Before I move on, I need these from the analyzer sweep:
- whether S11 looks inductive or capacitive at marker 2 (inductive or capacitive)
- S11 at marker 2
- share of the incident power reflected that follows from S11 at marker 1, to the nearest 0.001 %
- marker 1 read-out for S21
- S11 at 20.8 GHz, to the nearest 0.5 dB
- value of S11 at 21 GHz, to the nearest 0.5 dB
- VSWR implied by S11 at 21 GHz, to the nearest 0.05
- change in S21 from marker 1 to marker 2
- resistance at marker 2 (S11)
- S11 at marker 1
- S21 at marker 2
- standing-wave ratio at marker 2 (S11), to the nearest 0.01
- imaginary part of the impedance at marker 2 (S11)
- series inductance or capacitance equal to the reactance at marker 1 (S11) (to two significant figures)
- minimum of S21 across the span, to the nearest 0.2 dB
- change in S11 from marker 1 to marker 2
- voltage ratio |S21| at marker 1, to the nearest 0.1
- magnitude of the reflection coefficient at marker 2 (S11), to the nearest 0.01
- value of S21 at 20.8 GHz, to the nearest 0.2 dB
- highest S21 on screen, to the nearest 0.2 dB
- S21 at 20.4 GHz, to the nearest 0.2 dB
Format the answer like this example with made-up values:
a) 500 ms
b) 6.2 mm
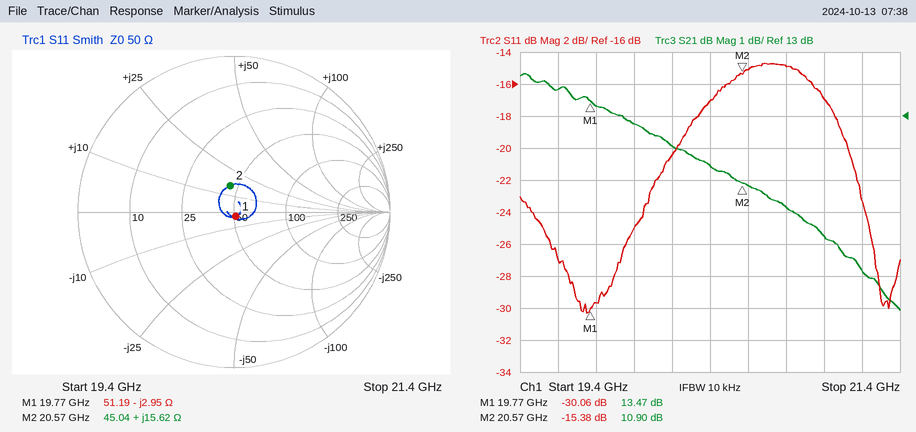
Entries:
a) inductive
b) -15.38 dB
c) 0.099 %
d) 13.47 dB
e) -15.0 dB
f) -17.0 dB
g) 1.35
h) -2.57 dB
i) 45.04 Ω
j) -30.06 dB
k) 10.90 dB
l) 1.41
m) +15.62 Ω
n) 2.7 pF
o) 7.0 dB
p) 14.68 dB
q) 4.7
r) 0.17
s) 10.2 dB
t) 14.4 dB
u) 11.4 dB
